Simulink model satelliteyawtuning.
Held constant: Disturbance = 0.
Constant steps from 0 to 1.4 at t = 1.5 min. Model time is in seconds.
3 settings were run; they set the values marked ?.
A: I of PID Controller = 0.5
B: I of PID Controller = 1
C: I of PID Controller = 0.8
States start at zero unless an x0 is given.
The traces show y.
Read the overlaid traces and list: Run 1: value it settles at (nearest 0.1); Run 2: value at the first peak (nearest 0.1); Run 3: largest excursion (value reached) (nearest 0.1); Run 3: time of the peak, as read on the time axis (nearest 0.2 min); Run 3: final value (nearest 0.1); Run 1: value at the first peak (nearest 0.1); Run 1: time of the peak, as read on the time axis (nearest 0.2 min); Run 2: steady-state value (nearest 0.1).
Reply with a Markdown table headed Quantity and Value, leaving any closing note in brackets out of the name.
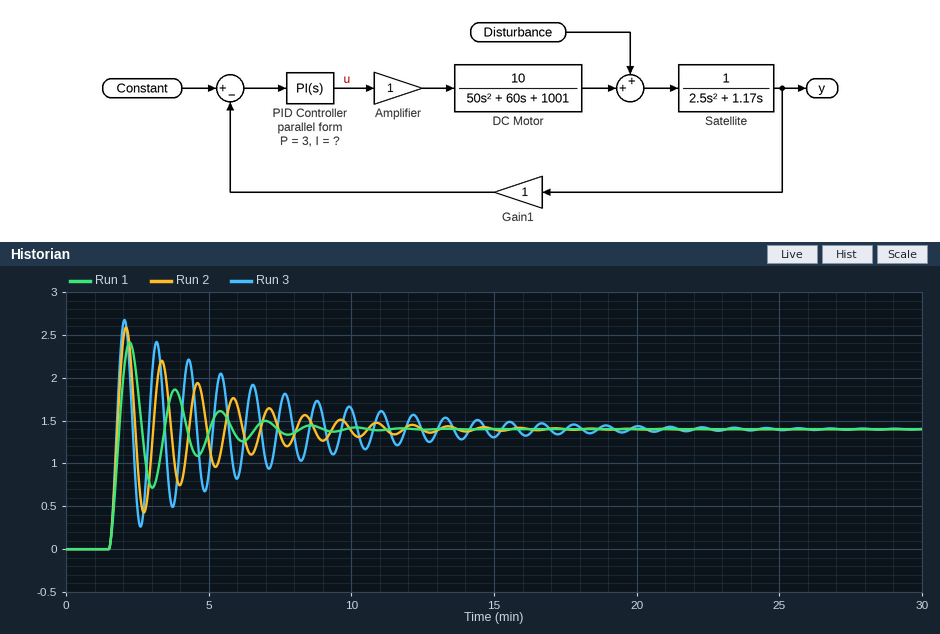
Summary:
| Quantity | Value |
|---|---|
| Run 1: value it settles at | 1.4 |
| Run 2: value at the first peak | 2.6 |
| Run 3: largest excursion (value reached) | 2.7 |
| Run 3: time of the peak, as read on the time axis | 2.0 min |
| Run 3: final value | 1.4 |
| Run 1: value at the first peak | 2.4 |
| Run 1: time of the peak, as read on the time axis | 2.2 min |
| Run 2: steady-state value | 1.4 |
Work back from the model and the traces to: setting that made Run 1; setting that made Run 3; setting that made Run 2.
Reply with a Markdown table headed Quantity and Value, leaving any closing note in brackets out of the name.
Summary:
| Quantity | Value |
|---|---|
| setting that made Run 1 | A |
| setting that made Run 3 | B |
| setting that made Run 2 | C |
